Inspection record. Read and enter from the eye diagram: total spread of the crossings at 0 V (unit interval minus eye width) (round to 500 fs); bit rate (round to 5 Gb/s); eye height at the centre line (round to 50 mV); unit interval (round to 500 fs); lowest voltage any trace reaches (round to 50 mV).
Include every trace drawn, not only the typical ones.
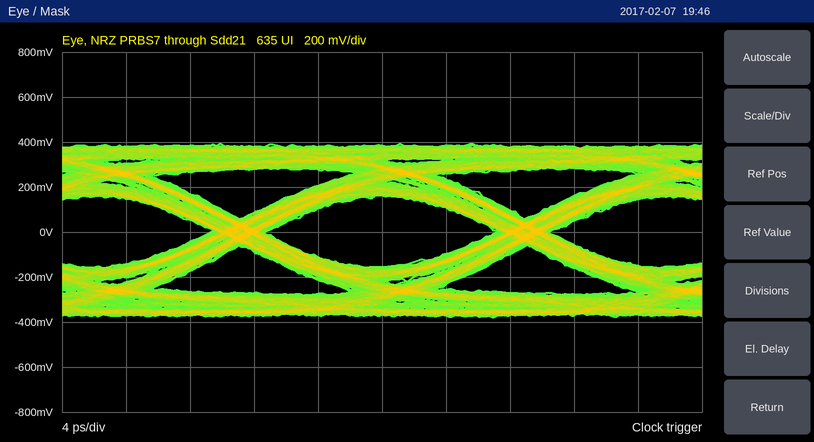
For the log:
3.5 ps
55 Gb/s
300 mV
18.0 ps
-400 mV
